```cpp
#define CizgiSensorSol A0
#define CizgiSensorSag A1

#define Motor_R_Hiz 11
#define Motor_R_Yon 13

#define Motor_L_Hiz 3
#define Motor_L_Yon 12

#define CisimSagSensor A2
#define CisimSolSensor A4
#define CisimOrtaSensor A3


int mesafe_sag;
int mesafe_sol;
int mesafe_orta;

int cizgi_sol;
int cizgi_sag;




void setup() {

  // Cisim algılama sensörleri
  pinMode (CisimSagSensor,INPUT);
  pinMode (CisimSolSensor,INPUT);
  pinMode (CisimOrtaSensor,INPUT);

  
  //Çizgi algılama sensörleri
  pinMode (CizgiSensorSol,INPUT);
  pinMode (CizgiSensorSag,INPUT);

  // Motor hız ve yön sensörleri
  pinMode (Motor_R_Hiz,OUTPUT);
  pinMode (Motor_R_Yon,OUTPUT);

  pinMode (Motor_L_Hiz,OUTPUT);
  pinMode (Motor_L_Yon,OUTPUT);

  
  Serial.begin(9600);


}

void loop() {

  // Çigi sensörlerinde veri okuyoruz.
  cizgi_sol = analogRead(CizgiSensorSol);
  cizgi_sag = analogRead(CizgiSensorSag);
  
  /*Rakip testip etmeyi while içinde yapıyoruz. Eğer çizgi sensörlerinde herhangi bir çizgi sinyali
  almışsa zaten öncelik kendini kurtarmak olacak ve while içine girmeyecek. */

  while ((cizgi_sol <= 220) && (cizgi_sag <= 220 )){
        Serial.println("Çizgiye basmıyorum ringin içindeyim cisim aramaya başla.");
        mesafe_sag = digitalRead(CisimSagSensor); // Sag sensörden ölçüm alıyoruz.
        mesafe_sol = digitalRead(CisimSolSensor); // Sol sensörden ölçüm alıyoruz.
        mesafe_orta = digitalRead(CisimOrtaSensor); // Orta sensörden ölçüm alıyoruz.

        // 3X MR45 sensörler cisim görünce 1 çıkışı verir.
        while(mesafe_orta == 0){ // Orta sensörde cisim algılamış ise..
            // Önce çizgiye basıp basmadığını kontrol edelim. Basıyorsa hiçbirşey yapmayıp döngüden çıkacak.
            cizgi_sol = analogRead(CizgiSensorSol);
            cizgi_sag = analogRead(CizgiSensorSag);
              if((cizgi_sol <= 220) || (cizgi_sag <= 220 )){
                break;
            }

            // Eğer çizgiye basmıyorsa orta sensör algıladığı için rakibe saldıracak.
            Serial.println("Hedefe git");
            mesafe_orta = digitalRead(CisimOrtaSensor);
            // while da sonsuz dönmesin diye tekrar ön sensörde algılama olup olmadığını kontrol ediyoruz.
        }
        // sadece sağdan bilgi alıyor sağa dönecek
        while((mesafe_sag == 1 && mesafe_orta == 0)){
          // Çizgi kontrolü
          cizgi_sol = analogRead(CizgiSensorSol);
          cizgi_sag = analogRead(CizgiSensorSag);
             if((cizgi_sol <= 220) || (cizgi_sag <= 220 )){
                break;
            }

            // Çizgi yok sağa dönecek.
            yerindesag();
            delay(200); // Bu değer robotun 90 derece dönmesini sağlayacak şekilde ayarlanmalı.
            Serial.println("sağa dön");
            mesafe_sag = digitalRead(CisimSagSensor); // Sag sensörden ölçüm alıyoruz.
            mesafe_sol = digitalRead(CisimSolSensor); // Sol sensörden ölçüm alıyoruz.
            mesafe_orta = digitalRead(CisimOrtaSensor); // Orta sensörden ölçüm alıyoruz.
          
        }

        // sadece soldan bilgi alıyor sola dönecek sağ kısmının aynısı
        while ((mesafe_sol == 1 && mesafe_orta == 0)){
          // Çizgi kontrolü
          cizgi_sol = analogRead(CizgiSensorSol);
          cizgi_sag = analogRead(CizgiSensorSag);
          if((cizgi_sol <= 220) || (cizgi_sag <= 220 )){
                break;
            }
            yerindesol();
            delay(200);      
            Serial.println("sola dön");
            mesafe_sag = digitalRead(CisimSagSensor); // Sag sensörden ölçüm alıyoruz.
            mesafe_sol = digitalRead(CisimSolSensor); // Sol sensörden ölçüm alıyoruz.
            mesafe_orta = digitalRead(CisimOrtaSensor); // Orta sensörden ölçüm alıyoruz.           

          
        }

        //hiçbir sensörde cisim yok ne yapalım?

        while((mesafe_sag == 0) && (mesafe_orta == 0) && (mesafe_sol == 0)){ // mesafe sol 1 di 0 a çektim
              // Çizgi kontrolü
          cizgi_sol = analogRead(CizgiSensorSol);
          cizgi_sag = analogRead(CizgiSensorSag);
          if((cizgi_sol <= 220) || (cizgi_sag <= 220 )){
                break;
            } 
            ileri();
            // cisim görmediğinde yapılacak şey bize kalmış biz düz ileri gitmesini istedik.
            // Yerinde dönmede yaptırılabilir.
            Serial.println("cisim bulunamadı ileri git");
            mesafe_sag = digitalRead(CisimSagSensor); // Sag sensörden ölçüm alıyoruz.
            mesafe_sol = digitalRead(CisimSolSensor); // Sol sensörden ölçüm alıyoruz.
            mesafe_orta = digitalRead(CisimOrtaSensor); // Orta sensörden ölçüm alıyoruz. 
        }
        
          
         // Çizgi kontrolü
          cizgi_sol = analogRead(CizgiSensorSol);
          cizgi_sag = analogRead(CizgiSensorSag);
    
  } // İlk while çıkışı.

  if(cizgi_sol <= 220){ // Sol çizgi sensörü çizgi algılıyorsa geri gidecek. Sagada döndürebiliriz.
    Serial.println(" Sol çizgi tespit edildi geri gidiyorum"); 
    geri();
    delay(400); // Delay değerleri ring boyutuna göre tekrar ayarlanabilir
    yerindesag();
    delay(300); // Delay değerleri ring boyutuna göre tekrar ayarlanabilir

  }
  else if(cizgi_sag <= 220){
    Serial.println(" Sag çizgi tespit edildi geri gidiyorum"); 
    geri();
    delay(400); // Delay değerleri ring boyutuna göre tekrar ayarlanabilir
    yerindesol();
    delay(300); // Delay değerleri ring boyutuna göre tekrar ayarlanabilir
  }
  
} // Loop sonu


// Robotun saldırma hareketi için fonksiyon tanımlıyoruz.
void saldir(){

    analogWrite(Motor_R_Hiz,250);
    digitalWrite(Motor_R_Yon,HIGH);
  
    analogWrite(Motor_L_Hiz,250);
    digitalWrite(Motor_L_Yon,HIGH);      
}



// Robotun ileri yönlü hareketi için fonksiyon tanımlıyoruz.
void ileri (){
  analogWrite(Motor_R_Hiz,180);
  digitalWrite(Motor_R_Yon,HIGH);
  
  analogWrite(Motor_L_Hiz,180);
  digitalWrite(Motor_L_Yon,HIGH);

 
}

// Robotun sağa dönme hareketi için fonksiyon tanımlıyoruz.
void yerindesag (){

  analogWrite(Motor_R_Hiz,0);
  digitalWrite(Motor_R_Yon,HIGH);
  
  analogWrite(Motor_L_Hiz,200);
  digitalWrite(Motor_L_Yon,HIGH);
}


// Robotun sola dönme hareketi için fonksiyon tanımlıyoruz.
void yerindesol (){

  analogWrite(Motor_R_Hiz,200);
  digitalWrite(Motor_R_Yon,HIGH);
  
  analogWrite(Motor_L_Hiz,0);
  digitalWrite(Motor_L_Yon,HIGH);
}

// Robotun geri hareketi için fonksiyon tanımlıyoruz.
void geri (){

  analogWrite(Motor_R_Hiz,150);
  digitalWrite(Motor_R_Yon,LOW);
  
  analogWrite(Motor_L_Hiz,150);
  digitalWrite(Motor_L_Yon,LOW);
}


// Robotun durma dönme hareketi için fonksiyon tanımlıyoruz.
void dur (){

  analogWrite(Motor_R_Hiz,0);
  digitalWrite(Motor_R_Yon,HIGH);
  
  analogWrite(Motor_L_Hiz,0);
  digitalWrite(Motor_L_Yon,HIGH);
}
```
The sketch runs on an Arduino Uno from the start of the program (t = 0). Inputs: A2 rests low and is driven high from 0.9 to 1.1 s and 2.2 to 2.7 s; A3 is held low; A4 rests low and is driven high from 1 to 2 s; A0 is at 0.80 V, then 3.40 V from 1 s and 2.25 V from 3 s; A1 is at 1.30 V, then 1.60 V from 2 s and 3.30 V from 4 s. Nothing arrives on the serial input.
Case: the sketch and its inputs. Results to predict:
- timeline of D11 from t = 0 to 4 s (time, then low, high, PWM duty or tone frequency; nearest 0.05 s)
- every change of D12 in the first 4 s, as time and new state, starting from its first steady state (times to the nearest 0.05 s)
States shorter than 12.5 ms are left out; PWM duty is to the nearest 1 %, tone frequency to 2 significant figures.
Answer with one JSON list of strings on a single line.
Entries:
["0 s PWM 59 %; 0.4 s low; 0.7 s PWM 59 %; 1.1 s low", "0 s low; 0.4 s high; 0.7 s low; 1.1 s high"]
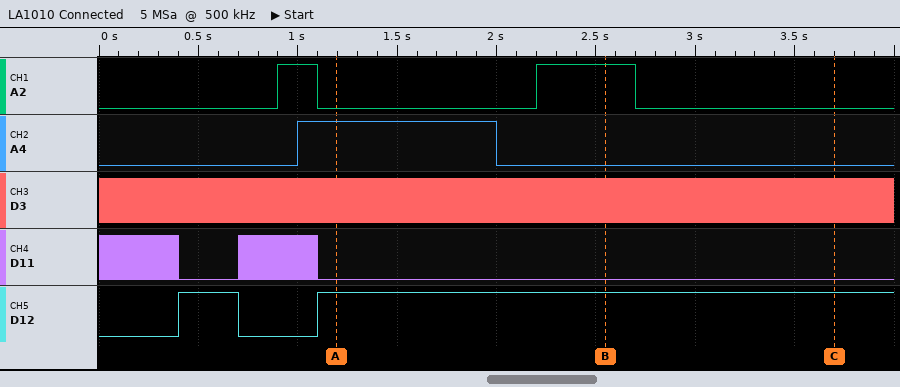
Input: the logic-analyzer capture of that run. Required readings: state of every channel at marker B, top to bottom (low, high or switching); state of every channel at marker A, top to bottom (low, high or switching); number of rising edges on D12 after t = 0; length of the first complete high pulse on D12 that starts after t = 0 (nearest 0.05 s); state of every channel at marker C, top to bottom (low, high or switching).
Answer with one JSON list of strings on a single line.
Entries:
["A2 high, A4 low, D3 switching, D11 low, D12 high", "A2 low, A4 high, D3 switching, D11 low, D12 high", "2", "0.30 s", "A2 low, A4 low, D3 switching, D11 low, D12 high"]
